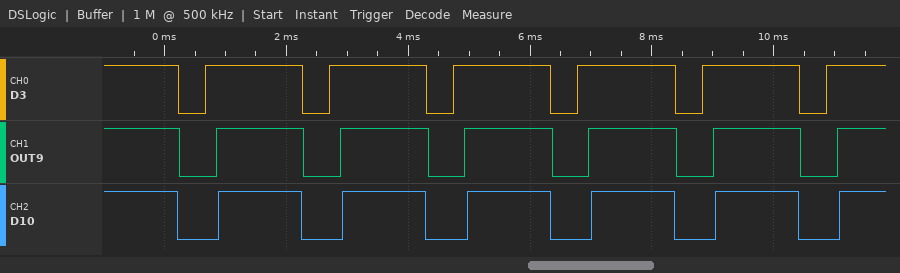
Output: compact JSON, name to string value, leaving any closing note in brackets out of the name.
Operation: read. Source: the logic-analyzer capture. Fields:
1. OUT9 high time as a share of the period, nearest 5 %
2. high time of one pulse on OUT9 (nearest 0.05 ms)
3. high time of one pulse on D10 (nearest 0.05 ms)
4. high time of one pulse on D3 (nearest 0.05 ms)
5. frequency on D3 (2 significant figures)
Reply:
{"OUT9 high time as a share of the period, nearest 5 %": "70 %", "high time of one pulse on OUT9": "1.45 ms", "high time of one pulse on D10": "1.35 ms", "high time of one pulse on D3": "1.60 ms", "frequency on D3": "490 Hz"}
